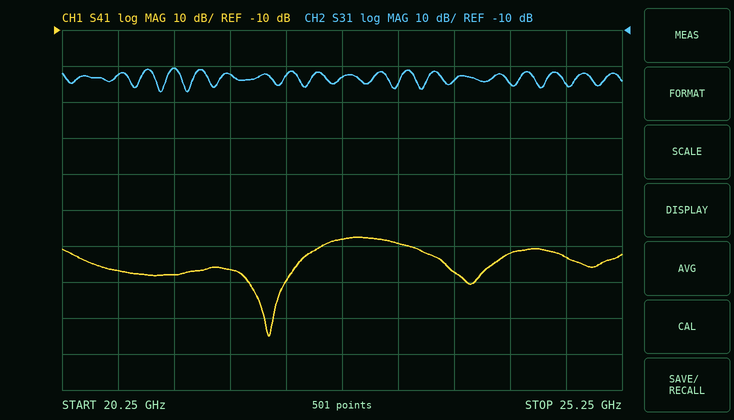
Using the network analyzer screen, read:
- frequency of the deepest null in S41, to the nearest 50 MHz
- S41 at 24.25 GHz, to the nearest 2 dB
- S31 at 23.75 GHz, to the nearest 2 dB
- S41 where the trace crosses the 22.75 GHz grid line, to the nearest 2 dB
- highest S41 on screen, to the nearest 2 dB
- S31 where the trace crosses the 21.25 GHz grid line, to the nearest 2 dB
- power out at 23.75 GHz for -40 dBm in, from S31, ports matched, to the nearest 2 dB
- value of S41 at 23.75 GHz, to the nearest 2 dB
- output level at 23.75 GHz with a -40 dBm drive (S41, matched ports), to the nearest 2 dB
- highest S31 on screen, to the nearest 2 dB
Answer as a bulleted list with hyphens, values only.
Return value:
- 22.10 GHz
- -72 dB
- -24 dB
- -68 dB
- -68 dB
- -20 dB
- -64 dBm
- -78 dB
- -118 dBm
- -20 dB
